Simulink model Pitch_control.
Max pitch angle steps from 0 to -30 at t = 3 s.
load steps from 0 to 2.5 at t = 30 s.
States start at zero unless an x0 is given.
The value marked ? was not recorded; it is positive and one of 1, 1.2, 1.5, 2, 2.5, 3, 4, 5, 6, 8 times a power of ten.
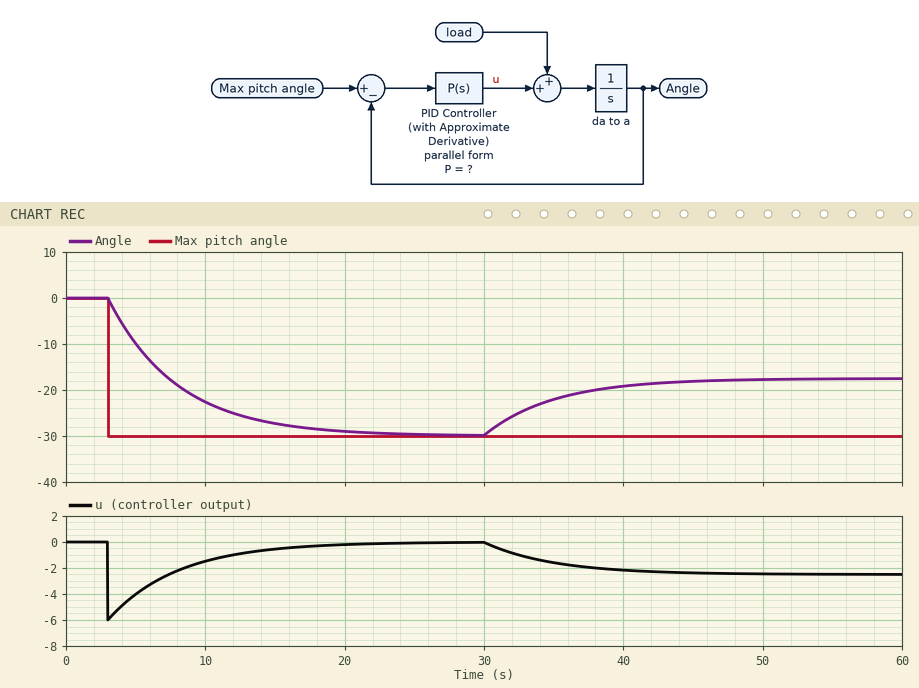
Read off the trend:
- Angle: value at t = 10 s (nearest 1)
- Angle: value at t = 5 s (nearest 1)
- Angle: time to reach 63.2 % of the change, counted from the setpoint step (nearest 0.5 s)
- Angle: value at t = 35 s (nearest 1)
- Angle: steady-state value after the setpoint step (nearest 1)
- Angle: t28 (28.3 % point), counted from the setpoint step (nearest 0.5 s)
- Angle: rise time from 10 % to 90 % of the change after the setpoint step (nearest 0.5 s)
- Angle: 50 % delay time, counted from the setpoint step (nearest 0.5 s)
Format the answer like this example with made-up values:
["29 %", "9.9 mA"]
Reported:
["-23", "-10", "5.0 s", "-22", "-30", "1.5 s", "11.0 s", "3.5 s"]
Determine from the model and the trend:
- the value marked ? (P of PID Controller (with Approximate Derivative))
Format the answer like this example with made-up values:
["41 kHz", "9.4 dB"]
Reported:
["0.2"]
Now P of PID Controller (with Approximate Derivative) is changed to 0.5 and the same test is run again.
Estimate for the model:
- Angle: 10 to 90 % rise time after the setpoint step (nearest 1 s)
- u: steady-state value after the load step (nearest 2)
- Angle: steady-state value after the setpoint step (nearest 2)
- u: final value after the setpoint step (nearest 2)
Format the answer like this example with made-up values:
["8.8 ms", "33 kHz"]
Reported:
["4 s", "-2", "-30", "0"]
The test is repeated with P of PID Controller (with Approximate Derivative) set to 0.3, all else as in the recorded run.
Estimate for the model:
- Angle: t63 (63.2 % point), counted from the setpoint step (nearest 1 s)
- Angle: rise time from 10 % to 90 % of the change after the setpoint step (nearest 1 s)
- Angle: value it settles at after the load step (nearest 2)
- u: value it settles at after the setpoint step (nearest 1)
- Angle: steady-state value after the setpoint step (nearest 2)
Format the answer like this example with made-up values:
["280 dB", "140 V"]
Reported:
["3 s", "7 s", "-22", "0", "-30"]
